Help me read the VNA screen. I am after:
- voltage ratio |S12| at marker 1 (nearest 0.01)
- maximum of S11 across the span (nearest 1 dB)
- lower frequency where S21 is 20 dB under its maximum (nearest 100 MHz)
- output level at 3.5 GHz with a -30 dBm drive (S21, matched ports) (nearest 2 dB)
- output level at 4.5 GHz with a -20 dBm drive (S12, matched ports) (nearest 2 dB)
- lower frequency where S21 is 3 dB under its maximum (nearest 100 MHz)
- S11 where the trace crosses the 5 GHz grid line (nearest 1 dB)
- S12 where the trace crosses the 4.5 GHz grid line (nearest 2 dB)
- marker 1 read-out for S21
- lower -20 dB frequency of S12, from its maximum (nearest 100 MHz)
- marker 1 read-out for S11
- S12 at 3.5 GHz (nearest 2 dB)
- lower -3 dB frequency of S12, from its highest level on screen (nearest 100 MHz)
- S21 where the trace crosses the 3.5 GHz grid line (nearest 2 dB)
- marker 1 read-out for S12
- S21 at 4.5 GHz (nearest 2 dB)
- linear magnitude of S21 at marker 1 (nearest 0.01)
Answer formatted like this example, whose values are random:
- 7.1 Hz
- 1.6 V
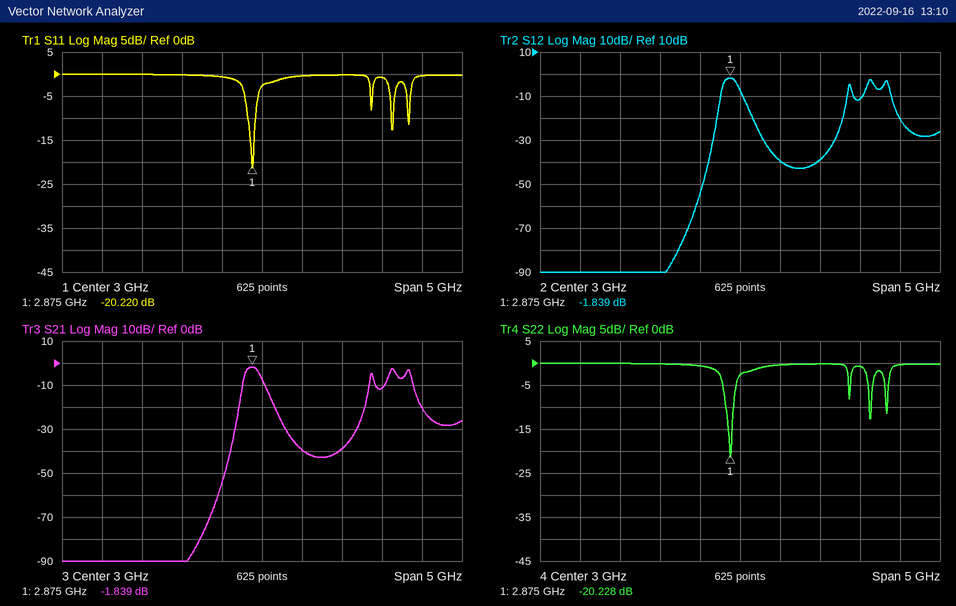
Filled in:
- 0.81
- 0 dB
- 2.7 GHz
- -70 dBm
- -32 dBm
- 2.8 GHz
- 0 dB
- -12 dB
- -1.839 dB
- 2.7 GHz
- -20.220 dB
- -40 dB
- 2.8 GHz
- -40 dB
- -1.839 dB
- -12 dB
- 0.81
